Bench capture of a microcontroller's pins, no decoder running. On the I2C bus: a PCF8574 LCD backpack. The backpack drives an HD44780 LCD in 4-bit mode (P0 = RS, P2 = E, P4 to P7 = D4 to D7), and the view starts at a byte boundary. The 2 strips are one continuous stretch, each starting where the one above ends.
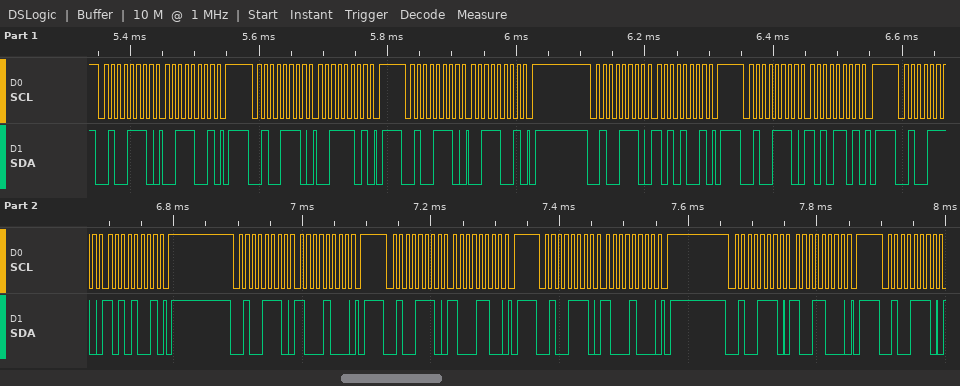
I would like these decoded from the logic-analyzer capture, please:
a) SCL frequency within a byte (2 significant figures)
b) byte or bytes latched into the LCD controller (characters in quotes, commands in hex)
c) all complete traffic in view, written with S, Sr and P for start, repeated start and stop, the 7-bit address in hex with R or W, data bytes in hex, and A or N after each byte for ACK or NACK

100 kHz
':'
S 27W A 39 A P S 27W A 3D A P S 27W A 39 A P S 27W A A9 A P S 27W A AD A P S 27W A A9 A P S 27W A 88 A P S 27W A 8C A P S 27W A 88 A P S 27W A 98 A P S 27W A
